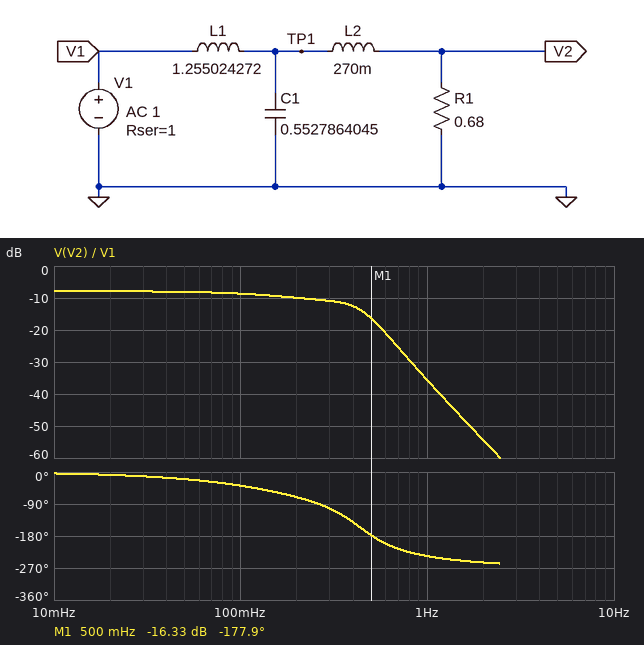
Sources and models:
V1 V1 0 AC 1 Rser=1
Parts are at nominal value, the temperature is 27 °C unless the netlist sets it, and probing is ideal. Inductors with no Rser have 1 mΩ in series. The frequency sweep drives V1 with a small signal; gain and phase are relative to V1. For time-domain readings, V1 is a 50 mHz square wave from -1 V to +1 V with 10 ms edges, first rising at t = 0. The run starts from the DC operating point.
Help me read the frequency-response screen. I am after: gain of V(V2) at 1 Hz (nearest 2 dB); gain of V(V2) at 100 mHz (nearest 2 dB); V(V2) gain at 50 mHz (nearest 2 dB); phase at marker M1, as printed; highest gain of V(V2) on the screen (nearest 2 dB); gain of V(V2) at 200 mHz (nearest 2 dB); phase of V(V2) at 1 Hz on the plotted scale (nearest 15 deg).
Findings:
-36 dB
-8 dB
-8 dB
-177.9 deg
-8 dB
-10 dB
-240 deg
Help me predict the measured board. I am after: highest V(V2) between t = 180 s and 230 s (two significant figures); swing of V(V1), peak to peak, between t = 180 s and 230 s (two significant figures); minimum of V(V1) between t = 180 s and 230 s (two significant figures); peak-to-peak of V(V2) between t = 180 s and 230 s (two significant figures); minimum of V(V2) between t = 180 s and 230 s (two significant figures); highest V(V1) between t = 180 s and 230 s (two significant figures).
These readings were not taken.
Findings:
400 mV
3.2 V
-1.6 V
810 mV
-400 mV
1.6 V
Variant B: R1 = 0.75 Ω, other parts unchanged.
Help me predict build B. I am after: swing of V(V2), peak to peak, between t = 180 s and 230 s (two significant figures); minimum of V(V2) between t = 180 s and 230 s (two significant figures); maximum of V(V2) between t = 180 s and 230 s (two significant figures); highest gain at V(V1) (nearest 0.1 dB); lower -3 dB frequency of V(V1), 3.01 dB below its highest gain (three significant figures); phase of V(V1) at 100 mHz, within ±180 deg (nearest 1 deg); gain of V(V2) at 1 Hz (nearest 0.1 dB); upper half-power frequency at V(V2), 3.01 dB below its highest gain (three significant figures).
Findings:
860 mV
-430 mV
430 mV
0 dB
198 mHz
21 deg
-35.0 dB
298 mHz
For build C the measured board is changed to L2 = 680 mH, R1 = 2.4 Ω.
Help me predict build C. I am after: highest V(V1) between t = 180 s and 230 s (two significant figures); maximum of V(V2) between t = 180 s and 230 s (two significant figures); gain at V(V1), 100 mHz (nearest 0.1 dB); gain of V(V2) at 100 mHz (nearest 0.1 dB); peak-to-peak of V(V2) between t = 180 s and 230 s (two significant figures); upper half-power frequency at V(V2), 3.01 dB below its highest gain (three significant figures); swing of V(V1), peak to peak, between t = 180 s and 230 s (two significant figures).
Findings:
1.3 V
910 mV
-3.9 dB
-2.6 dB
1.8 V
283 mHz
2.6 V
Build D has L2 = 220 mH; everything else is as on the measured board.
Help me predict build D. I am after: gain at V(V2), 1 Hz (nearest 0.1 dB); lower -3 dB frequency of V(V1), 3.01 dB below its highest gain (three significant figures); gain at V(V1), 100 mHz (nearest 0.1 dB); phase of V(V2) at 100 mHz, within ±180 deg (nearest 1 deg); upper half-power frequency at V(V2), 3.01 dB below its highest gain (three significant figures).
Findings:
-34.0 dB
190 mHz
-5.1 dB
-38 deg
265 mHz
